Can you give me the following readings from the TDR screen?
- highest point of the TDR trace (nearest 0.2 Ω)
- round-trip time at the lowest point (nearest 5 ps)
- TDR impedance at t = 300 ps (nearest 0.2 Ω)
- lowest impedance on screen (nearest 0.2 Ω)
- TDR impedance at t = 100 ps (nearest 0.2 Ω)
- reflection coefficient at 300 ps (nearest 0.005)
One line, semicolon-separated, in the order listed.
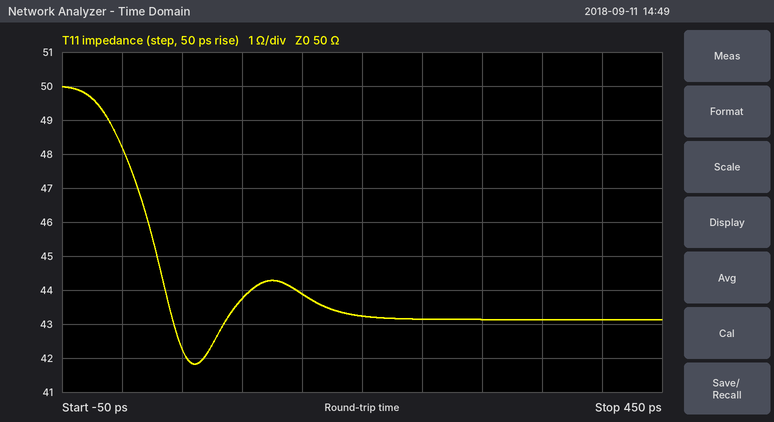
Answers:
50.0 Ω; 60 ps; 43.2 Ω; 41.8 Ω; 43.8 Ω; -0.075
